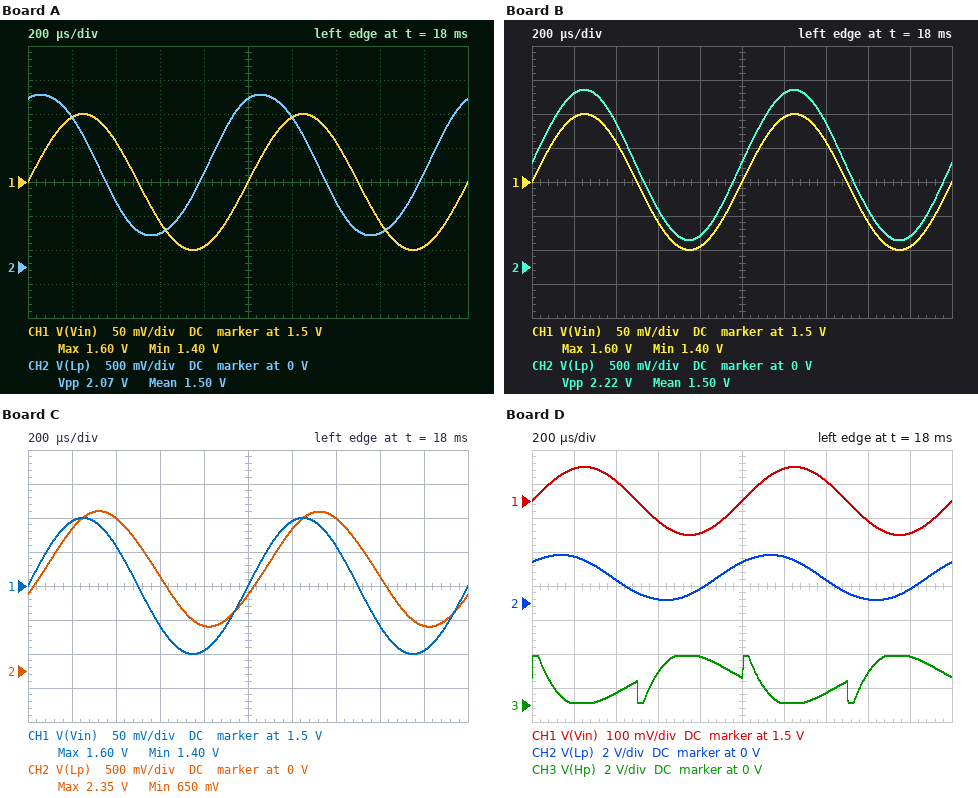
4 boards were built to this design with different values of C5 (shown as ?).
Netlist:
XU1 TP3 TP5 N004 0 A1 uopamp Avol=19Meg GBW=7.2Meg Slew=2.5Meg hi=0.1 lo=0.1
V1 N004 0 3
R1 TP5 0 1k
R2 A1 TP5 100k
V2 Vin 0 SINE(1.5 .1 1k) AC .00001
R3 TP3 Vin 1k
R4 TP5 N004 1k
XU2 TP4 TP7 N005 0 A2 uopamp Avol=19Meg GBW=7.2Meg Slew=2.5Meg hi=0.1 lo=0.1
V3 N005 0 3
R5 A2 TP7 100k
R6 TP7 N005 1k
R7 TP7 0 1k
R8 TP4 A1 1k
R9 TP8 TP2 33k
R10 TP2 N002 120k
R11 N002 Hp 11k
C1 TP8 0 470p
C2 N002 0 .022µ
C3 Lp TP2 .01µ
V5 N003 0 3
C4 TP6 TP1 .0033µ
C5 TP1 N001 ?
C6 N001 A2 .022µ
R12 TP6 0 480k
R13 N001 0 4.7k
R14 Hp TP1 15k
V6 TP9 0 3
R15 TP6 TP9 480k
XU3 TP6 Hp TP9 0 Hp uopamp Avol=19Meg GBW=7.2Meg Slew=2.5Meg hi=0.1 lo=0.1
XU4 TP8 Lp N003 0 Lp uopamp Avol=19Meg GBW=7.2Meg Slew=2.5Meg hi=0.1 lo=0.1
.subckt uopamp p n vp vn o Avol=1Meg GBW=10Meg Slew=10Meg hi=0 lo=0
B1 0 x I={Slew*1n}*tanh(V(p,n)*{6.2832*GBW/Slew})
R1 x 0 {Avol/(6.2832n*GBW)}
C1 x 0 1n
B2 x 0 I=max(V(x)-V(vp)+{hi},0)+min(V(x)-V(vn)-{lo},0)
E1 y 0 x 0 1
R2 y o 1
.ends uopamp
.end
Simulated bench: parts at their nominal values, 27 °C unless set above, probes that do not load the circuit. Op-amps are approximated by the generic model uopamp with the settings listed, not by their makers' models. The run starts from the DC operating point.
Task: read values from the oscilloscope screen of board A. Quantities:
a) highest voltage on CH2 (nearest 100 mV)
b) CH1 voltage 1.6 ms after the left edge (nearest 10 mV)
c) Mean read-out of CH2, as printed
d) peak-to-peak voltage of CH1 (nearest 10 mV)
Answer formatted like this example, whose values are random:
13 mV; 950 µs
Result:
2.5 V; 1.44 V; 1.50 V; 200 mV
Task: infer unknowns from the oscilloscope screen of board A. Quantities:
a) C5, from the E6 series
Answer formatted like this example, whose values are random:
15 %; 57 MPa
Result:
1.5 nF
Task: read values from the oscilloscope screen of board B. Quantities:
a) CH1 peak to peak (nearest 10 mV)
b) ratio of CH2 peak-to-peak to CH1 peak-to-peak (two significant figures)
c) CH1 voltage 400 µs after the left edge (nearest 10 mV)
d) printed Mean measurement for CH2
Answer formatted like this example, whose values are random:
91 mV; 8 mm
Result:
200 mV; 11; 1.56 V; 1.50 V
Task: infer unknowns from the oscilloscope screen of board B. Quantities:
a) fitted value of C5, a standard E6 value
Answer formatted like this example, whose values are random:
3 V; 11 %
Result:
4.7 nF
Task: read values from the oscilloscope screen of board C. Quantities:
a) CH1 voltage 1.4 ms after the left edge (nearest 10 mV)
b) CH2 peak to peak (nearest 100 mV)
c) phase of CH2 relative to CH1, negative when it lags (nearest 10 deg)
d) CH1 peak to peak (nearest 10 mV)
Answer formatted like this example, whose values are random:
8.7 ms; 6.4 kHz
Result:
1.56 V; 1.7 V; -30 deg; 200 mV
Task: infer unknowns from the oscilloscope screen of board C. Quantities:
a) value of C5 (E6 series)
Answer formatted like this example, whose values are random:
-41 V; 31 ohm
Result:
10 nF
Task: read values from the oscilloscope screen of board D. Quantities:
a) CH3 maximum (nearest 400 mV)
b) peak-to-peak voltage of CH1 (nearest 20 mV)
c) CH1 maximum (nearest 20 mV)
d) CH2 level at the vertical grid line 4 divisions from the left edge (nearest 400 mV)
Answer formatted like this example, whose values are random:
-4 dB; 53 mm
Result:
2.8 V; 200 mV; 1.60 V; 800 mV
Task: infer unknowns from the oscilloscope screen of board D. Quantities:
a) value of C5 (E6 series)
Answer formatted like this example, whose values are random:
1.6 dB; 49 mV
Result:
2.2 nF
